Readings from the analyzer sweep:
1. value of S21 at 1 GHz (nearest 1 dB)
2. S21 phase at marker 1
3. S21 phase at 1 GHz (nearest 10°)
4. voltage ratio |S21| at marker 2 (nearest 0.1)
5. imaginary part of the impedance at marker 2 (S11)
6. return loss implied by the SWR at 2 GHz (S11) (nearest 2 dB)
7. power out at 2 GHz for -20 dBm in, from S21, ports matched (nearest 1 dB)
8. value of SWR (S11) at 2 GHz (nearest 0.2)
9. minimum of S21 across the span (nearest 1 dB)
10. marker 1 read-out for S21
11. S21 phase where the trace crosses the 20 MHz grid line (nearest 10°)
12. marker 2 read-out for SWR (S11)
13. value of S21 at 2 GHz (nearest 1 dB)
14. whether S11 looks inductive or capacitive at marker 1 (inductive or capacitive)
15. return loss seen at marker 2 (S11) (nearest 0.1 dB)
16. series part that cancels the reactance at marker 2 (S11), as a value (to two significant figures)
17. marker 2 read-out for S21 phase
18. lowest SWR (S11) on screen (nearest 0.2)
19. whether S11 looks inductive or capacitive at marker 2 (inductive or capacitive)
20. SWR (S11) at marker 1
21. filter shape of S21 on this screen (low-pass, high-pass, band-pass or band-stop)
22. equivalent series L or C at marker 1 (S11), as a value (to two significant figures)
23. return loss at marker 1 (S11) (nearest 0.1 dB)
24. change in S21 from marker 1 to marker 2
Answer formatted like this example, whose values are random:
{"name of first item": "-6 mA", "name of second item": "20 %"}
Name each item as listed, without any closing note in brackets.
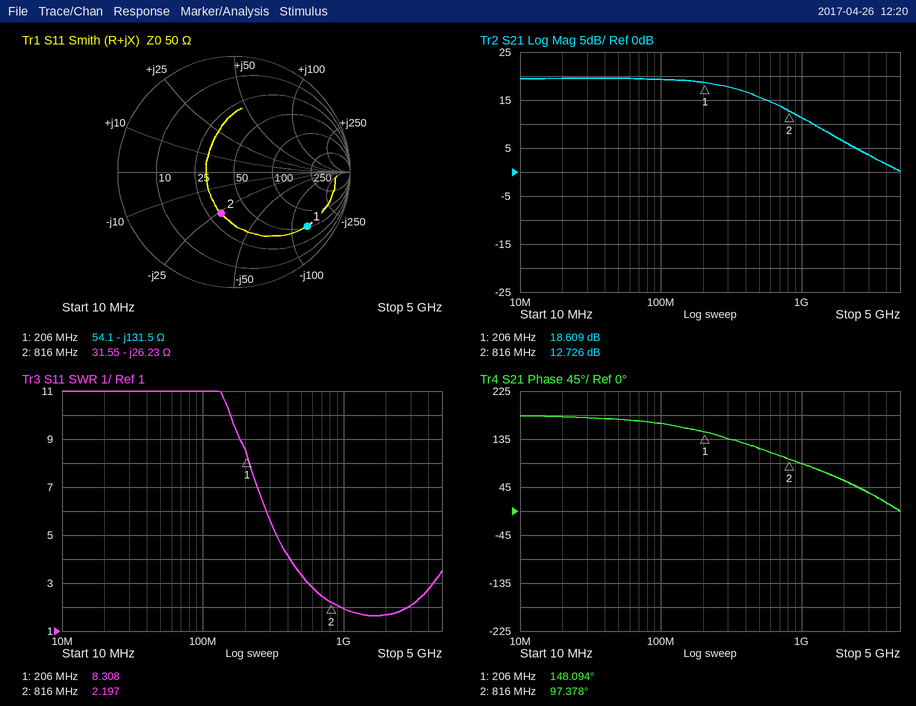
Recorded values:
{"value of S21 at 1 GHz": "11 dB", "S21 phase at marker 1": "148.094°", "S21 phase at 1 GHz": "90°", "voltage ratio |S21| at marker 2": "4.3", "imaginary part of the impedance at marker 2": "-26.23 Ω", "return loss implied by the SWR at 2 GHz (S11)": "12 dB", "power out at 2 GHz for -20 dBm in, from S21, ports matched": "-14 dBm", "value of SWR (S11) at 2 GHz": "1.6", "minimum of S21 across the span": "0 dB", "marker 1 read-out for S21": "18.609 dB", "S21 phase where the trace crosses the 20 MHz grid line": "180°", "marker 2 read-out for SWR": "2.197", "value of S21 at 2 GHz": "6 dB", "whether S11 looks inductive or capacitive at marker 1": "capacitive", "return loss seen at marker 2 (S11)": "8.5 dB", "series part that cancels the reactance at marker 2 (S11), as a value": "5.1 nH", "marker 2 read-out for S21 phase": "97.378°", "lowest SWR (S11) on screen": "1.6", "whether S11 looks inductive or capacitive at marker 2": "capacitive", "SWR (S11) at marker 1": "8.308", "filter shape of S21 on this screen": "low-pass", "equivalent series L or C at marker 1 (S11), as a value": "5.9 pF", "return loss at marker 1 (S11)": "2.1 dB", "change in S21 from marker 1 to marker 2": "-5.883 dB"}
